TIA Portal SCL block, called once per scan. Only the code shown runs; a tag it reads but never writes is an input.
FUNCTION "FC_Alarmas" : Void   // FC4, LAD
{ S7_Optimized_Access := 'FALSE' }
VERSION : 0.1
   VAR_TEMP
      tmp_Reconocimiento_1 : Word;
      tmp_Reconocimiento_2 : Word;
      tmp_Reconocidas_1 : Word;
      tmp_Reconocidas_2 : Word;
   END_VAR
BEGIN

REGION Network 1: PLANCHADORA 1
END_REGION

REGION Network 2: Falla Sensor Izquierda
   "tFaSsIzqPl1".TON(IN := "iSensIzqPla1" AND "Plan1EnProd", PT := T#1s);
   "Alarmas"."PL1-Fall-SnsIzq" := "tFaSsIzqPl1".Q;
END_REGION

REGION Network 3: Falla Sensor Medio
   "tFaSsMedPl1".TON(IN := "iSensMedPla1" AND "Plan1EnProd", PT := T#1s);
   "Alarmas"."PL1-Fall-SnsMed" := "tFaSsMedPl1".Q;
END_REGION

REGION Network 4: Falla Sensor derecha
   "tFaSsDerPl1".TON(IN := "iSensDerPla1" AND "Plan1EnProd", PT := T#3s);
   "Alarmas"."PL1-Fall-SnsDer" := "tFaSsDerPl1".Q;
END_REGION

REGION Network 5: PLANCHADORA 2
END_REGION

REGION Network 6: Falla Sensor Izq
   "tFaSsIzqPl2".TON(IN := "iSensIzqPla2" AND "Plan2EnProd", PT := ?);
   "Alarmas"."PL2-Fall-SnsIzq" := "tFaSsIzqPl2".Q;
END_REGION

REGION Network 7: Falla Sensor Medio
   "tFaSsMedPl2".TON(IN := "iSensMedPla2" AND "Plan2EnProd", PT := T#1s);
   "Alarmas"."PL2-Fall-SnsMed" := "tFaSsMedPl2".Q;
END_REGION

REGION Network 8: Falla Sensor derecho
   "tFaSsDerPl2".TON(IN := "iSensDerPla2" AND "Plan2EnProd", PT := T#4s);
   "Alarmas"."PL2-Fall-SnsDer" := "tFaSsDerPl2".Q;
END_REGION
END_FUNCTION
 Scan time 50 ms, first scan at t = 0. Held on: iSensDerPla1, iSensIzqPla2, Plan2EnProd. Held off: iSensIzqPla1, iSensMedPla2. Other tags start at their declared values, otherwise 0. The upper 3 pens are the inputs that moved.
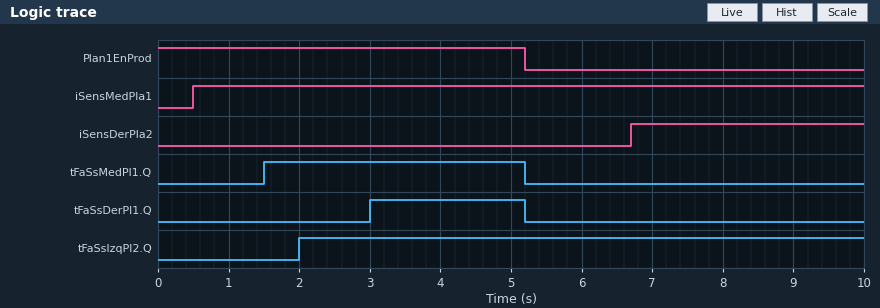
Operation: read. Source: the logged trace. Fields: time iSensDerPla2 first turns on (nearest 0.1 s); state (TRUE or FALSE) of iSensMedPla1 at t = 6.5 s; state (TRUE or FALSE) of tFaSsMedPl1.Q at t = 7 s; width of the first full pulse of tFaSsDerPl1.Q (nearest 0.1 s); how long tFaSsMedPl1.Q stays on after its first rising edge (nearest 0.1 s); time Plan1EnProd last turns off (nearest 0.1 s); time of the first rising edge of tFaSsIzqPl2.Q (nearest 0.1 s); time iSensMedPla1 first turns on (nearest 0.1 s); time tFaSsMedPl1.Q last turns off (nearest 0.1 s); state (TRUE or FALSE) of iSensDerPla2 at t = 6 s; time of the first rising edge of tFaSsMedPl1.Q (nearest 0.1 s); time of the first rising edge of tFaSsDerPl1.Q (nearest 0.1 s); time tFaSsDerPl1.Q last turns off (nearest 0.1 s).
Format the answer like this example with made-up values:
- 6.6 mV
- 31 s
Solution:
- 6.7 s
- TRUE
- FALSE
- 2.2 s
- 3.7 s
- 5.2 s
- 2.0 s
- 0.5 s
- 5.2 s
- FALSE
- 1.5 s
- 3.0 s
- 5.2 s
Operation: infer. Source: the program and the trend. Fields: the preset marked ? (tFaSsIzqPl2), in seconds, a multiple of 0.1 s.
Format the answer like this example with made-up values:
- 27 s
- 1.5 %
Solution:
- 2.0 s
